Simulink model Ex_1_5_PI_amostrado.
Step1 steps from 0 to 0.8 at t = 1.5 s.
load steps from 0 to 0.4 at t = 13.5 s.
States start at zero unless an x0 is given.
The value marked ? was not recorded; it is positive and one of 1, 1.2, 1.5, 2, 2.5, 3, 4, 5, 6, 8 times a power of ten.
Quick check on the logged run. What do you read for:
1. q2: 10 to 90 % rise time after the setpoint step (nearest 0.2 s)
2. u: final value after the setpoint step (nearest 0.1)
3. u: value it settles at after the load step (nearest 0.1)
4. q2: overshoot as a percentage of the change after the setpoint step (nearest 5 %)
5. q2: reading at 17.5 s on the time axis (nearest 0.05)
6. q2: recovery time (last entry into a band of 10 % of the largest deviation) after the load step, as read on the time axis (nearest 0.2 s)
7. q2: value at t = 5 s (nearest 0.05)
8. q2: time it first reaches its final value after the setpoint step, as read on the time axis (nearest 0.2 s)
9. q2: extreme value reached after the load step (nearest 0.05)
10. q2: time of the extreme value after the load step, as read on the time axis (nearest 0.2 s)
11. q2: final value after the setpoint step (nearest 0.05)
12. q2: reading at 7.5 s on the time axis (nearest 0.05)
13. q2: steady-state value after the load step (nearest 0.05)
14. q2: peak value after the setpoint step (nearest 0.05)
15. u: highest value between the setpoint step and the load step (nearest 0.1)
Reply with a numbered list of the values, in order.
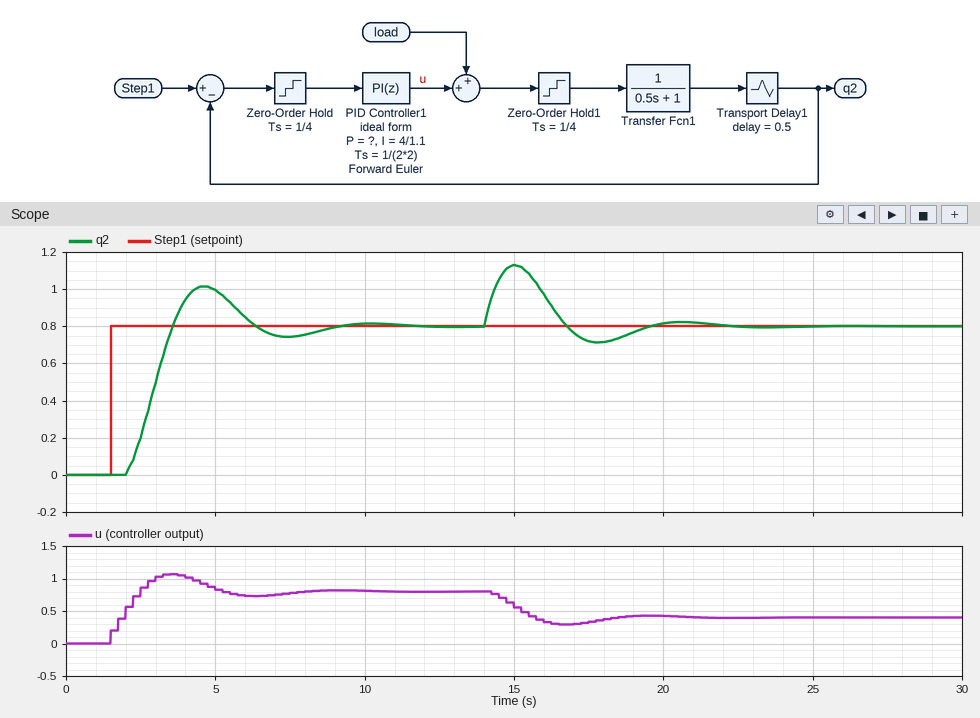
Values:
1. 1.2 s
2. 0.8
3. 0.4
4. 25 %
5. 0.70
6. 19.0 s
7. 1.00
8. 3.6 s
9. 1.15
10. 15.0 s
11. 0.80
12. 0.75
13. 0.80
14. 1.00
15. 1.1
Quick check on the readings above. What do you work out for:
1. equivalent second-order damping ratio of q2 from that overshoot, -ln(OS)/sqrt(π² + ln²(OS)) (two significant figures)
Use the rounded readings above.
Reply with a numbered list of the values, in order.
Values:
1. 0.40
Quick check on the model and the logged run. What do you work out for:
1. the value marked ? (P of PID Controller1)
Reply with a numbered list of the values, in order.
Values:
1. 0.25
